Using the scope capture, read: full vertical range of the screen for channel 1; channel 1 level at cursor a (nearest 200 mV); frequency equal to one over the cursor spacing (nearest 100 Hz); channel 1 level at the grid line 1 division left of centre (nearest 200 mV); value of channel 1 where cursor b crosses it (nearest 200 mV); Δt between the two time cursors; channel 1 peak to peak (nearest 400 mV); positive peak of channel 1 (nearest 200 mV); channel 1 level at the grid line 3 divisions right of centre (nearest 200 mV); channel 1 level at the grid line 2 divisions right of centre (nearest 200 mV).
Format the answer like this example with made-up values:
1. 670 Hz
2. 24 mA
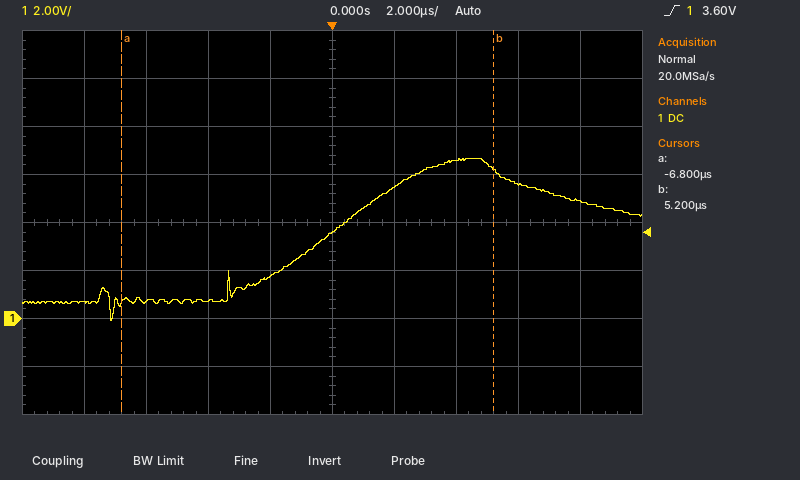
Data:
1. 16 V
2. 600 mV
3. 83.3 kHz
4. 1.8 V
5. 6.2 V
6. 12.0 µs
7. 6.8 V
8. 6.6 V
9. 5.6 V
10. 6.6 V
